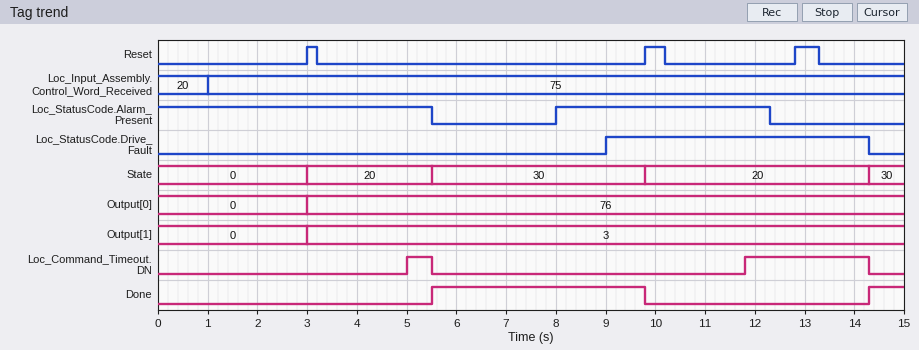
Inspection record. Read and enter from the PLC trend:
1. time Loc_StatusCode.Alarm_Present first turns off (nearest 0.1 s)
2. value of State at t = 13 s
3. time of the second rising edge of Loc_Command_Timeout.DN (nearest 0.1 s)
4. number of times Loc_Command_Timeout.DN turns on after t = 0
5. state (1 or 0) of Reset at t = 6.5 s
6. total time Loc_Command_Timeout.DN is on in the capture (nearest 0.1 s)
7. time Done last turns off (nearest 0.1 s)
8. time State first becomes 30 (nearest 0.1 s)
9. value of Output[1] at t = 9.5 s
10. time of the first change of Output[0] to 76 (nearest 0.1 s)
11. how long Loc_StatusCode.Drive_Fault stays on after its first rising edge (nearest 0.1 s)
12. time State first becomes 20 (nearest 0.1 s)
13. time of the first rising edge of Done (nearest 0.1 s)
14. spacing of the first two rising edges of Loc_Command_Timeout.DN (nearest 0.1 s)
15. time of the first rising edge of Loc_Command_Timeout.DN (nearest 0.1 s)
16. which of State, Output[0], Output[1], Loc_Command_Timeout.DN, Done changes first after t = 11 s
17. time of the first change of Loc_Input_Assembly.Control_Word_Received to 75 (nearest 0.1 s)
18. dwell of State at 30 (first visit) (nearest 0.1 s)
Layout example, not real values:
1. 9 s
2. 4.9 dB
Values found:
1. 5.5 s
2. 20
3. 11.8 s
4. 2
5. 0
6. 3.0 s
7. 9.8 s
8. 5.5 s
9. 3
10. 3.0 s
11. 5.3 s
12. 3.0 s
13. 5.5 s
14. 6.8 s
15. 5.0 s
16. Loc_Command_Timeout.DN
17. 1.0 s
18. 4.3 s
